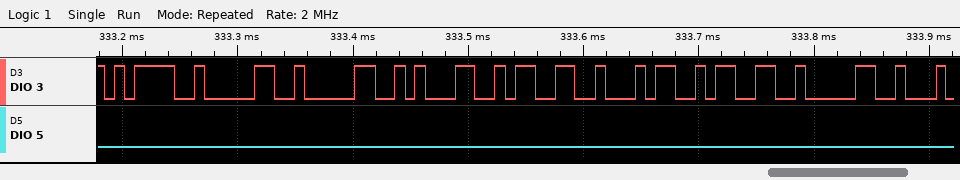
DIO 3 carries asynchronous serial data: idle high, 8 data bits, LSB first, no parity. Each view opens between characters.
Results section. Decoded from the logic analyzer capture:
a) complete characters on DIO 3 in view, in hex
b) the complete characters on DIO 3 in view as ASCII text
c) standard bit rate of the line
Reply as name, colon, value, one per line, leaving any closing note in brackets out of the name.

complete characters on DIO 3 in view, in hex: 3D, 30, 30, 31, 33, 34, 33, 30
the complete characters on DIO 3 in view as ASCII text: "=0013430"
standard bit rate of the line: 115200 baud
